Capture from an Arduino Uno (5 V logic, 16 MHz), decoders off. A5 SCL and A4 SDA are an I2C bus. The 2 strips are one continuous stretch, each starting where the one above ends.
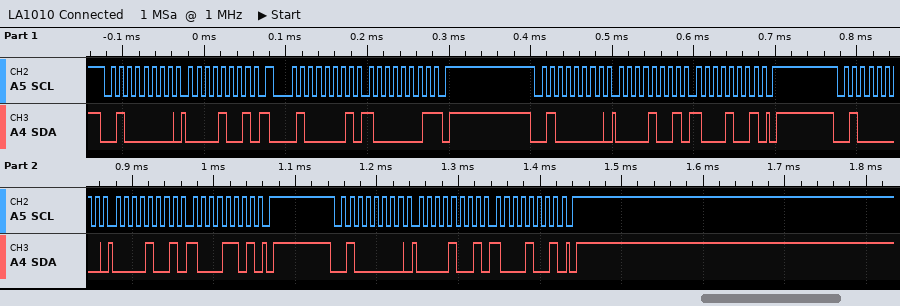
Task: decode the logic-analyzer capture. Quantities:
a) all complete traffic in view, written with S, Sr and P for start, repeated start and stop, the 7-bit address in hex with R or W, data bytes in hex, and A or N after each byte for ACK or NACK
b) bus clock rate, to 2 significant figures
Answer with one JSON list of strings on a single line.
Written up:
["S 20W A 09 A Sr 20R A 81 N P S 20W A 09 A 89 A P S 20W A 09 A 8D A P S 20W A 09 A 89 A P", "100 kHz"]
